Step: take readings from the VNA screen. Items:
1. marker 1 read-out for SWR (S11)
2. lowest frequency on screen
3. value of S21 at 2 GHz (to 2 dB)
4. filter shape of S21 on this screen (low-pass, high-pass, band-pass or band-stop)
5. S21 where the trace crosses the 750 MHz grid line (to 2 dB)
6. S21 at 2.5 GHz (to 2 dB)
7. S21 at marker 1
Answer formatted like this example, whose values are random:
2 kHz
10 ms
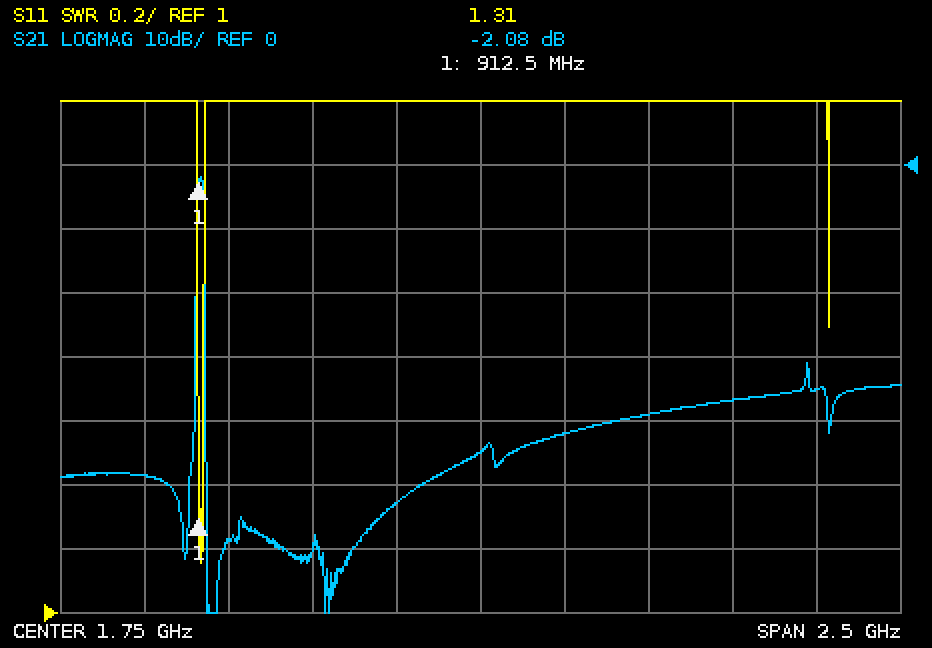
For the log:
1.31
500 MHz
-42 dB
band-pass
-48 dB
-36 dB
-2.08 dB
